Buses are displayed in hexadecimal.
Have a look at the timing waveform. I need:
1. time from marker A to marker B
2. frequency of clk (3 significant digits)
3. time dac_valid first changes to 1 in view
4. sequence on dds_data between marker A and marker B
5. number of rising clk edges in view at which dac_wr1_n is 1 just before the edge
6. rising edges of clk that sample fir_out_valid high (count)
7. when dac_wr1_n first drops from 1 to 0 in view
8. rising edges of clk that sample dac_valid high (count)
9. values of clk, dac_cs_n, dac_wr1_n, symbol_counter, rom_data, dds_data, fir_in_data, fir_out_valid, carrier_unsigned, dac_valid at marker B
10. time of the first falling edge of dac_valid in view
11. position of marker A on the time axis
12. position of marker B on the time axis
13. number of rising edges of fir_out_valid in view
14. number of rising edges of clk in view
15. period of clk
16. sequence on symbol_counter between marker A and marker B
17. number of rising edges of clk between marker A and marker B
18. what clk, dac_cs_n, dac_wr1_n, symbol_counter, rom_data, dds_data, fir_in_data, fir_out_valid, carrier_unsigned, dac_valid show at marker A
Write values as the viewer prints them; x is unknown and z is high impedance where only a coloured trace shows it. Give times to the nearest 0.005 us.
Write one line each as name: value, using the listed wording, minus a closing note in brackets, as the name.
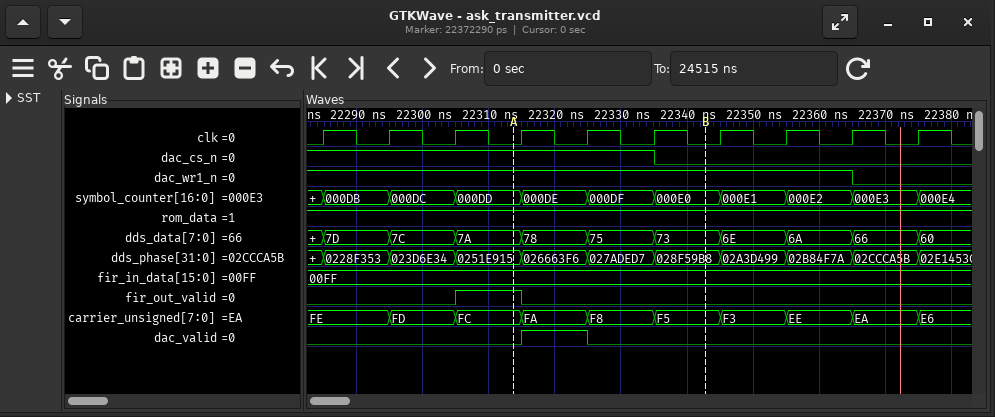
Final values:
time from marker A to marker B: 0.03 us
frequency of clk: 100 MHz
time dac_valid first changes to 1 in view: 22.315 us
sequence on dds_data between marker A and marker B: 7A, 78, 75, 73
number of rising clk edges in view at which dac_wr1_n is 1 just before the edge: 9
rising edges of clk that sample fir_out_valid high: 1
when dac_wr1_n first drops from 1 to 0 in view: 22.365 us
rising edges of clk that sample dac_valid high: 1
values of clk, dac_cs_n, dac_wr1_n, symbol_counter, rom_data, dds_data, fir_in_data, fir_out_valid, carrier_unsigned, dac_valid at marker B: clk=0, dac_cs_n=0, dac_wr1_n=1, symbol_counter=000E0, rom_data=1, dds_data=73, fir_in_data=00FF, fir_out_valid=0, carrier_unsigned=F5, dac_valid=0
time of the first falling edge of dac_valid in view: 22.325 us
position of marker A on the time axis: 22.315 us
position of marker B on the time axis: 22.345 us
number of rising edges of fir_out_valid in view: 1
number of rising edges of clk in view: 10
period of clk: 0.01 us
sequence on symbol_counter between marker A and marker B: 000DD, 000DE, 000DF, 000E0
number of rising edges of clk between marker A and marker B: 3
what clk, dac_cs_n, dac_wr1_n, symbol_counter, rom_data, dds_data, fir_in_data, fir_out_valid, carrier_unsigned, dac_valid show at marker A: clk=0, dac_cs_n=1, dac_wr1_n=1, symbol_counter=000DD, rom_data=1, dds_data=7A, fir_in_data=00FF, fir_out_valid=1, carrier_unsigned=FC, dac_valid=0
